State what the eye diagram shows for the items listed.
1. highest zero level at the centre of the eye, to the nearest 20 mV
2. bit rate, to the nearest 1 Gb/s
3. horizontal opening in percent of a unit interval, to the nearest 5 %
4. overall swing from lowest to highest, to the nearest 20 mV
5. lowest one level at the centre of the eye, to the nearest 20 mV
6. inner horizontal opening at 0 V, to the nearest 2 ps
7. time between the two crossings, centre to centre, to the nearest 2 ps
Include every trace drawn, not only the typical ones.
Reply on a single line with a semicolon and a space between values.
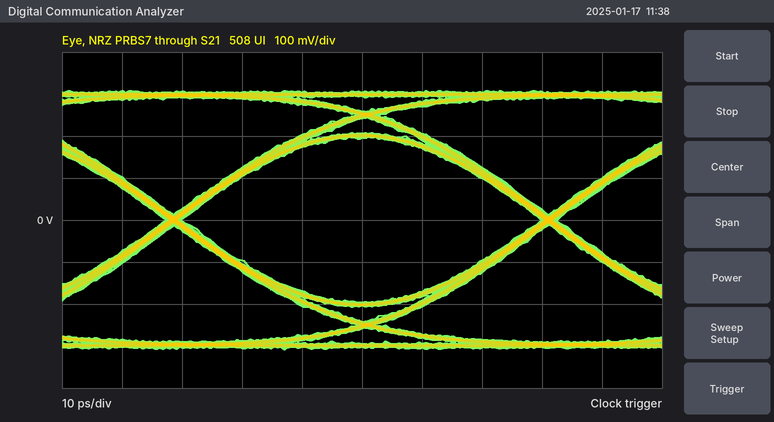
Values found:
-200 mV; 16 Gb/s; 95 %; 620 mV; 200 mV; 60 ps; 62 ps
